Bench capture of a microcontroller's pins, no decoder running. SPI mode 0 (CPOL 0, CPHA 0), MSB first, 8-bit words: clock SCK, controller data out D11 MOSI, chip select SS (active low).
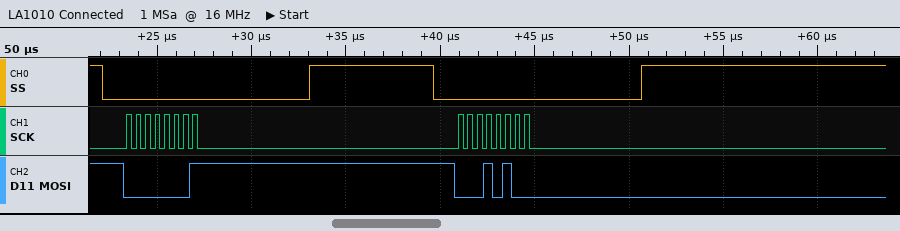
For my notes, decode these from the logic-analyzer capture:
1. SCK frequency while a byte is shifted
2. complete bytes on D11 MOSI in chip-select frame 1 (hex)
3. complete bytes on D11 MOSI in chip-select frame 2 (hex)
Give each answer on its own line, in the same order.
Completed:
2 MHz
01
14
